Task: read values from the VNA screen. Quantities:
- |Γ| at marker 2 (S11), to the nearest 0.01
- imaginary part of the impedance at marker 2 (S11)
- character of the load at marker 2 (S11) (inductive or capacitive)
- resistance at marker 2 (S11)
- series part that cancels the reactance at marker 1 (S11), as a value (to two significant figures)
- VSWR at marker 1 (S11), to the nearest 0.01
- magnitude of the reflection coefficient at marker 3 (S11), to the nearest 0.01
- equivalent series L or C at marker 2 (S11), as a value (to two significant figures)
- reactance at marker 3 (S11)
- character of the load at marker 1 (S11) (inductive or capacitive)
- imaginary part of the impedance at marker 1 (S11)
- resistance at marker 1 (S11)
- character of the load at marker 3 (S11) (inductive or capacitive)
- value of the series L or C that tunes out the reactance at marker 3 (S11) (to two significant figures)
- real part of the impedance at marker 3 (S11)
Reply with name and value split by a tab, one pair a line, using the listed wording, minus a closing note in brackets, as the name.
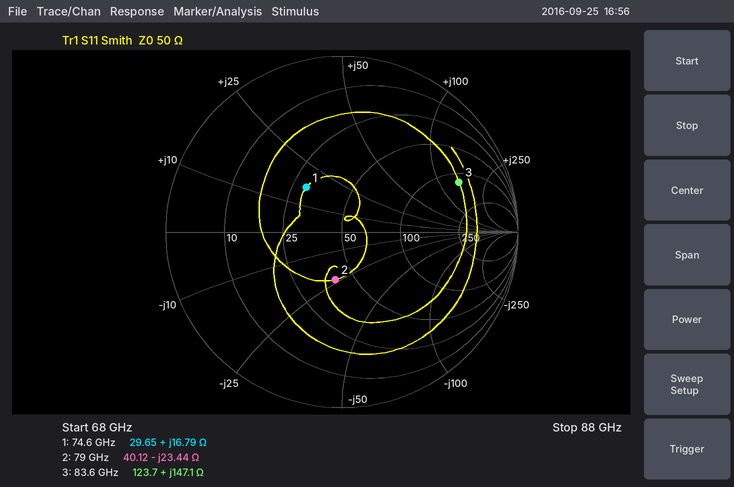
|Γ| at marker 2 (S11), to the nearest 0.01	0.27
imaginary part of the impedance at marker 2	-23.44 Ω
character of the load at marker 2 (S11)	capacitive
resistance at marker 2	40.12 Ω
series part that cancels the reactance at marker 1 (S11), as a value	130 fF
VSWR at marker 1 (S11), to the nearest 0.01	1.96
magnitude of the reflection coefficient at marker 3 (S11), to the nearest 0.01	0.72
equivalent series L or C at marker 2 (S11), as a value	86 fF
reactance at marker 3	+147.1 Ω
character of the load at marker 1 (S11)	inductive
imaginary part of the impedance at marker 1	+16.79 Ω
resistance at marker 1	29.65 Ω
character of the load at marker 3 (S11)	inductive
value of the series L or C that tunes out the reactance at marker 3 (S11)	13 fF
real part of the impedance at marker 3	123.7 Ω
